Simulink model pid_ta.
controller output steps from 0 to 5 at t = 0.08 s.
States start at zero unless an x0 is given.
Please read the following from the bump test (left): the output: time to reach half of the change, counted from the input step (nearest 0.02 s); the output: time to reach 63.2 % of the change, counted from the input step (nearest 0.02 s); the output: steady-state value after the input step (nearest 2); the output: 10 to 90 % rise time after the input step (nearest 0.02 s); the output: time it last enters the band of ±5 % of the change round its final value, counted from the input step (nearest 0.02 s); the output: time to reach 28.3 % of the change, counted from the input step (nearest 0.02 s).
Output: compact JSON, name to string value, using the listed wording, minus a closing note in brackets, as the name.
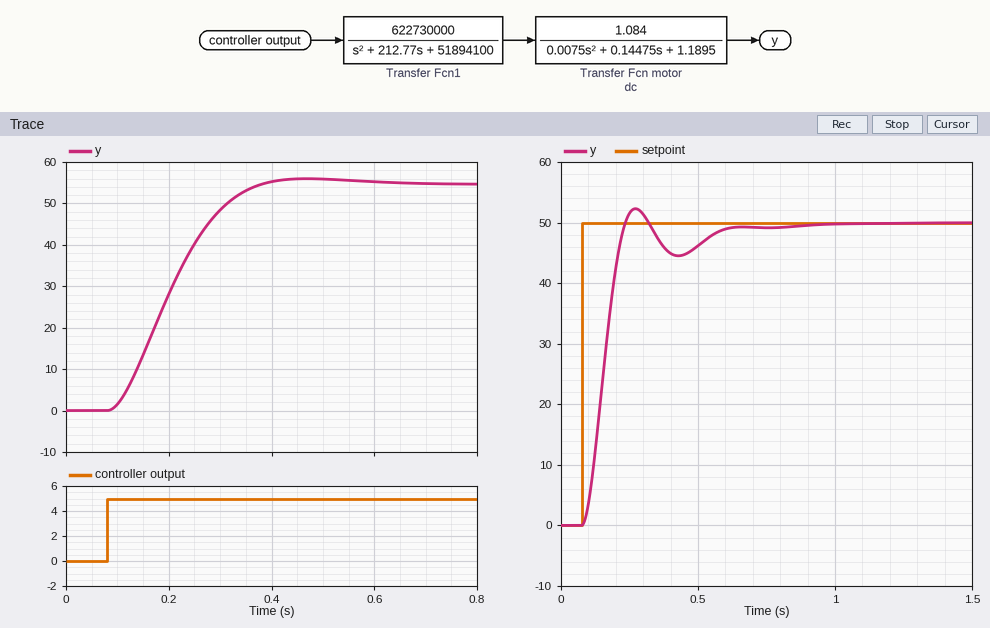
{"the output: time to reach half of the change, counted from the input step": "0.12 s", "the output: time to reach 63.2 % of the change, counted from the input step": "0.14 s", "the output: steady-state value after the input step": "54", "the output: 10 to 90 % rise time after the input step": "0.18 s", "the output: time it last enters the band of ±5 % of the change round its final value, counted from the input step": "0.26 s", "the output: time to reach 28.3 % of the change, counted from the input step": "0.08 s"}
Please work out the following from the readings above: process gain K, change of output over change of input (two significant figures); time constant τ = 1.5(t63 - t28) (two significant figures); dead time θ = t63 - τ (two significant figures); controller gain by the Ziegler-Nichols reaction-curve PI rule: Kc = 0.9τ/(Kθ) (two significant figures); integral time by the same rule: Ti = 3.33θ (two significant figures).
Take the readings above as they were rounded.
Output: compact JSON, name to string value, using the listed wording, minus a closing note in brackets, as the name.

{"process gain K, change of output over change of input": "11", "time constant τ = 1.5(t63 - t28)": "0.090 s", "dead time θ = t63 - τ": "0.050 s", "controller gain by the Ziegler-Nichols reaction-curve PI rule: Kc = 0.9τ/(Kθ)": "0.15", "integral time by the same rule: Ti = 3.33θ": "0.17 s"}
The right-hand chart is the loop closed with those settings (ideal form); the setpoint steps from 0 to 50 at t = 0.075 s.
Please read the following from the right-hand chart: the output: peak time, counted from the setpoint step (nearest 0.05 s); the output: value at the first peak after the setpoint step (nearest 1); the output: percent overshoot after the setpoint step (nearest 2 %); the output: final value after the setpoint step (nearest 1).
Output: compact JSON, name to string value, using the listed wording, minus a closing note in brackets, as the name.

{"the output: peak time, counted from the setpoint step": "0.20 s", "the output: value at the first peak after the setpoint step": "52", "the output: percent overshoot after the setpoint step": "4 %", "the output: final value after the setpoint step": "50"}
